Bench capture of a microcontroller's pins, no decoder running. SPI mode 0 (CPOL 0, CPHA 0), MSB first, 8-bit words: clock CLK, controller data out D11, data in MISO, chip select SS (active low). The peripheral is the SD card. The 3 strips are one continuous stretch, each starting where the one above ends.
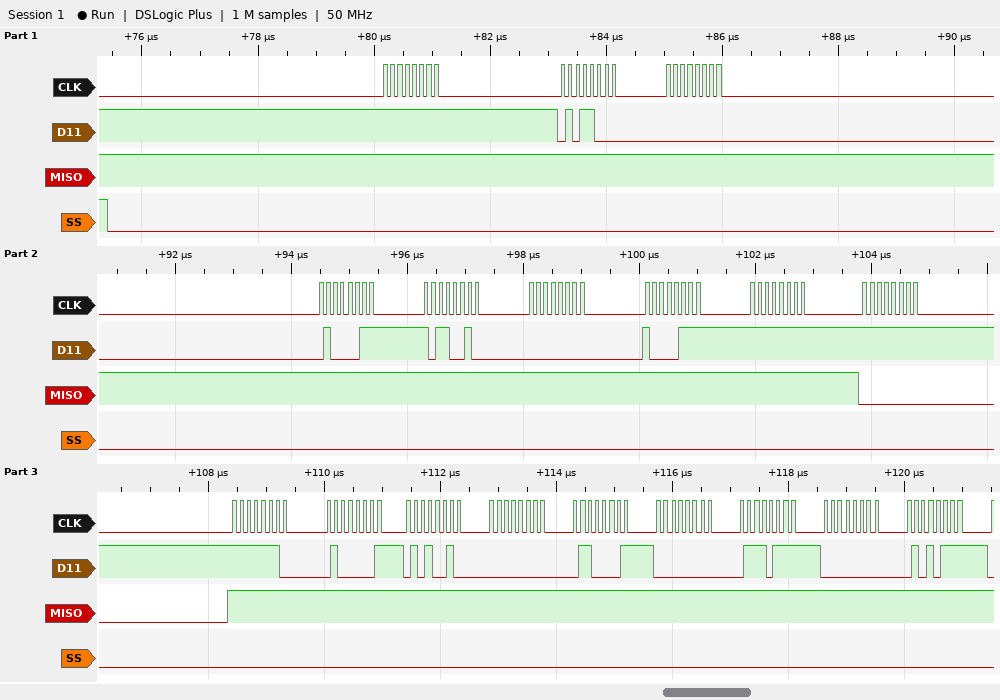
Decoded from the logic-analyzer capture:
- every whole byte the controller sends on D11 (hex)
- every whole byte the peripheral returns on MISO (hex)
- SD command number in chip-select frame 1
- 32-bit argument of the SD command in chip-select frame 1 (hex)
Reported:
FF 58 00 43 B2 00 87 FF FF FE 41 52 00 61 00 77 00 57
FF FF FF FF FF FF FF FF 00 FF FF FF FF FF FF FF FF FF
CMD24
0x0043B200
